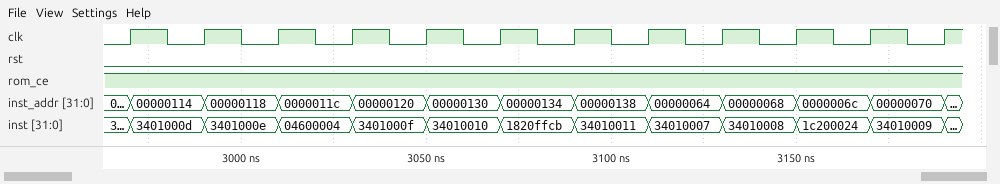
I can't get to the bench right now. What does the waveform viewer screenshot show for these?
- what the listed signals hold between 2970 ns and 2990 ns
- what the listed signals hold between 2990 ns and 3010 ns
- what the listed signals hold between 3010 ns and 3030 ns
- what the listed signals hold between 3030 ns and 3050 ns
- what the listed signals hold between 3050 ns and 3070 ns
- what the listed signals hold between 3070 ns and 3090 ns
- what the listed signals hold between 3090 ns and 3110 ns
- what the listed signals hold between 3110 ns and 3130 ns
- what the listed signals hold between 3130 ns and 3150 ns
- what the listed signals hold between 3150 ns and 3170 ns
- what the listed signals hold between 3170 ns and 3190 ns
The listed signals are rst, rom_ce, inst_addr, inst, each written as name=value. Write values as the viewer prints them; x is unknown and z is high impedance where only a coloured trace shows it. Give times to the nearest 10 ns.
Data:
rst=0, rom_ce=1, inst_addr=00000114, inst=3401000d
rst=0, rom_ce=1, inst_addr=00000118, inst=3401000e
rst=0, rom_ce=1, inst_addr=0000011c, inst=04600004
rst=0, rom_ce=1, inst_addr=00000120, inst=3401000f
rst=0, rom_ce=1, inst_addr=00000130, inst=34010010
rst=0, rom_ce=1, inst_addr=00000134, inst=1820ffcb
rst=0, rom_ce=1, inst_addr=00000138, inst=34010011
rst=0, rom_ce=1, inst_addr=00000064, inst=34010007
rst=0, rom_ce=1, inst_addr=00000068, inst=34010008
rst=0, rom_ce=1, inst_addr=0000006c, inst=1c200024
rst=0, rom_ce=1, inst_addr=00000070, inst=34010009
